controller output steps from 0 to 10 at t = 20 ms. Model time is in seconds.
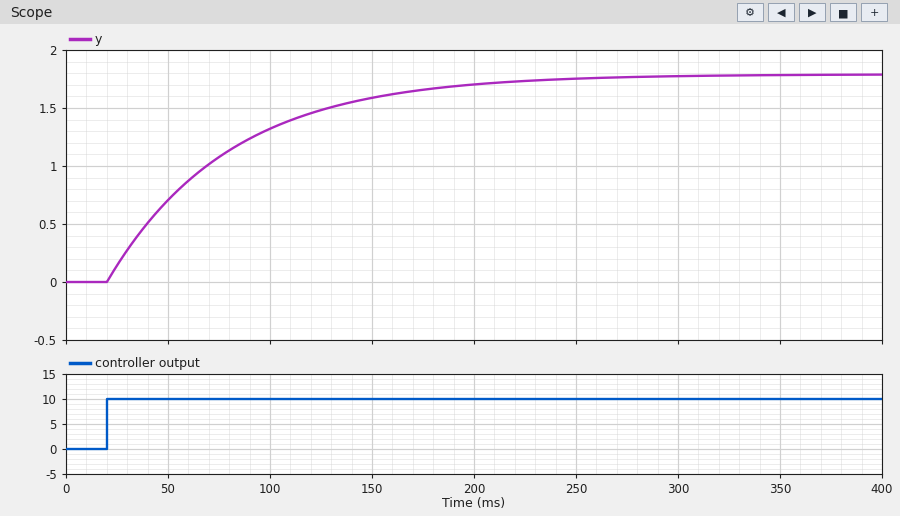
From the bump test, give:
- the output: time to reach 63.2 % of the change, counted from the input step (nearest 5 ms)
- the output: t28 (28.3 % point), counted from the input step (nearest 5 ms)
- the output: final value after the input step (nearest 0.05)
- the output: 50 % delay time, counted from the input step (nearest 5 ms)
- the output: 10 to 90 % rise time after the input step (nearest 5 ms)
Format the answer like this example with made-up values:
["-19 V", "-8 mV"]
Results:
["60 ms", "20 ms", "1.80", "40 ms", "130 ms"]
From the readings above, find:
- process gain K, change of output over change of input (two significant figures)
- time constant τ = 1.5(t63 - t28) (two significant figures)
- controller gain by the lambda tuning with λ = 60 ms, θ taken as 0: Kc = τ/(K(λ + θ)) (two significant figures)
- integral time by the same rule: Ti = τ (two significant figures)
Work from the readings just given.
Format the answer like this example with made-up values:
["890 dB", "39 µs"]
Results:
["0.18", "60 ms", "5.6", "60 ms"]
